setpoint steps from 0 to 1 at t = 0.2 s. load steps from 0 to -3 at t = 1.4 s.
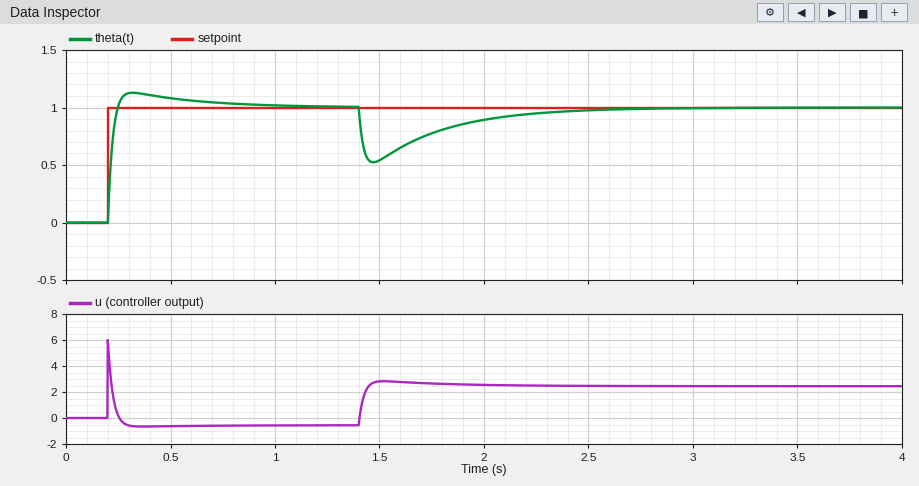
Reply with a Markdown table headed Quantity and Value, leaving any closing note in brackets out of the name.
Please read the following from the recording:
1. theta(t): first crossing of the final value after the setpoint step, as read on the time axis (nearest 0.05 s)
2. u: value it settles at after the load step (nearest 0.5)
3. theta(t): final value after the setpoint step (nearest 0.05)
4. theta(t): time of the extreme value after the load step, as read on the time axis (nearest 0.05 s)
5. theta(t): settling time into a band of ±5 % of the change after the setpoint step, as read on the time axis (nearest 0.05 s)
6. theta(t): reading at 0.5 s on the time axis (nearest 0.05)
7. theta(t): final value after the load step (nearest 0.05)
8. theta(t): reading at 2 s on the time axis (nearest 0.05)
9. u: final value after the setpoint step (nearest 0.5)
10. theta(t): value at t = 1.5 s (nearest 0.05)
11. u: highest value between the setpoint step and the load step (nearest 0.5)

| Quantity | Value |
|---|---|
| theta(t): first crossing of the final value after the setpoint step, as read on the time axis | 0.25 s |
| u: value it settles at after the load step | 2.5 |
| theta(t): final value after the setpoint step | 1.00 |
| theta(t): time of the extreme value after the load step, as read on the time axis | 1.45 s |
| theta(t): settling time into a band of ±5 % of the change after the setpoint step, as read on the time axis | 0.65 s |
| theta(t): reading at 0.5 s on the time axis | 1.10 |
| theta(t): final value after the load step | 1.00 |
| theta(t): reading at 2 s on the time axis | 0.90 |
| u: final value after the setpoint step | -0.5 |
| theta(t): value at t = 1.5 s | 0.55 |
| u: highest value between the setpoint step and the load step | 6.0 |
